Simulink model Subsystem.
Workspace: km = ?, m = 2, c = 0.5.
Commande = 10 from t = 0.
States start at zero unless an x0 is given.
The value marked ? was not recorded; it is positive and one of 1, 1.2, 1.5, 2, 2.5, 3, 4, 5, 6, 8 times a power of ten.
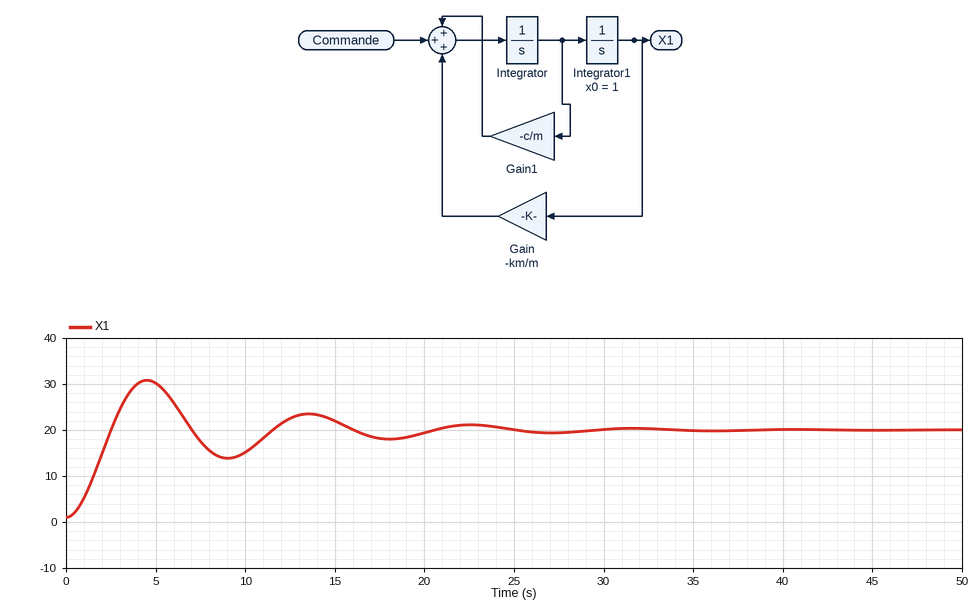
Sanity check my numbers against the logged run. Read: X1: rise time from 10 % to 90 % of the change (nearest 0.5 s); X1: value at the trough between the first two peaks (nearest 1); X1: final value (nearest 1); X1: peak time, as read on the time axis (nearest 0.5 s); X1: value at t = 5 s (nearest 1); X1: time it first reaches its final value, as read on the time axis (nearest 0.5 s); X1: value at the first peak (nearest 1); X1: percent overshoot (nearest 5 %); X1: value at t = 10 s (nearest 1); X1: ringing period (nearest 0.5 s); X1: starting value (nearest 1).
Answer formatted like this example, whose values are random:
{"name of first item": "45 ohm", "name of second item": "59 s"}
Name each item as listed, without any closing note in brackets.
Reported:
{"X1: rise time from 10 % to 90 % of the change": "1.5 s", "X1: value at the trough between the first two peaks": "14", "X1: final value": "20", "X1: peak time, as read on the time axis": "4.5 s", "X1: value at t = 5 s": "30", "X1: time it first reaches its final value, as read on the time axis": "2.5 s", "X1: value at the first peak": "31", "X1: percent overshoot": "55 %", "X1: value at t = 10 s": "15", "X1: ringing period": "9.0 s", "X1: starting value": "1"}
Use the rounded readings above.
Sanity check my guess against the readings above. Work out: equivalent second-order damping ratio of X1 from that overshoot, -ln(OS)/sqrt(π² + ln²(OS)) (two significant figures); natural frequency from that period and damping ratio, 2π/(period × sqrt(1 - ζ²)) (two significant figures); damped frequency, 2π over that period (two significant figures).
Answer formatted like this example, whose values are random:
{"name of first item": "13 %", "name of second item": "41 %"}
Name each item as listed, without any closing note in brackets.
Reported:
{"equivalent second-order damping ratio of X1 from that overshoot, -ln(OS)/sqrt(π² + ln²(OS))": "0.19", "natural frequency from that period and damping ratio, 2π/(period × sqrt(1 - ζ²))": "0.71 rad/s", "damped frequency, 2π over that period": "0.70 rad/s"}
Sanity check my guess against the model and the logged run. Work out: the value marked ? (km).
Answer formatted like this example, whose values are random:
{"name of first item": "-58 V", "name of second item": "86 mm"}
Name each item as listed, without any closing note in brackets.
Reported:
{"the value marked ?": "1"}
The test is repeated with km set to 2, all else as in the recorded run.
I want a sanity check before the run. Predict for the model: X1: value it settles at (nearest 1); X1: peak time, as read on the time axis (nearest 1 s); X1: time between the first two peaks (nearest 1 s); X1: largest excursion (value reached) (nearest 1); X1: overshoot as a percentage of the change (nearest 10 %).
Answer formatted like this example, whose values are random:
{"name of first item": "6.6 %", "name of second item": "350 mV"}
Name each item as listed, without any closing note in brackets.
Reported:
{"X1: value it settles at": "10", "X1: peak time, as read on the time axis": "3 s", "X1: time between the first two peaks": "6 s", "X1: largest excursion (value reached)": "16", "X1: overshoot as a percentage of the change": "70 %"}
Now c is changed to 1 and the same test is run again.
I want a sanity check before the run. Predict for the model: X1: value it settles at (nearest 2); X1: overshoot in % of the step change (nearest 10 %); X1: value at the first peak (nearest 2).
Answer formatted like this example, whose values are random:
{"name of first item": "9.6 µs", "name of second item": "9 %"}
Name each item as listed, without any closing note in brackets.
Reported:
{"X1: value it settles at": "20", "X1: overshoot in % of the step change": "30 %", "X1: value at the first peak": "26"}
